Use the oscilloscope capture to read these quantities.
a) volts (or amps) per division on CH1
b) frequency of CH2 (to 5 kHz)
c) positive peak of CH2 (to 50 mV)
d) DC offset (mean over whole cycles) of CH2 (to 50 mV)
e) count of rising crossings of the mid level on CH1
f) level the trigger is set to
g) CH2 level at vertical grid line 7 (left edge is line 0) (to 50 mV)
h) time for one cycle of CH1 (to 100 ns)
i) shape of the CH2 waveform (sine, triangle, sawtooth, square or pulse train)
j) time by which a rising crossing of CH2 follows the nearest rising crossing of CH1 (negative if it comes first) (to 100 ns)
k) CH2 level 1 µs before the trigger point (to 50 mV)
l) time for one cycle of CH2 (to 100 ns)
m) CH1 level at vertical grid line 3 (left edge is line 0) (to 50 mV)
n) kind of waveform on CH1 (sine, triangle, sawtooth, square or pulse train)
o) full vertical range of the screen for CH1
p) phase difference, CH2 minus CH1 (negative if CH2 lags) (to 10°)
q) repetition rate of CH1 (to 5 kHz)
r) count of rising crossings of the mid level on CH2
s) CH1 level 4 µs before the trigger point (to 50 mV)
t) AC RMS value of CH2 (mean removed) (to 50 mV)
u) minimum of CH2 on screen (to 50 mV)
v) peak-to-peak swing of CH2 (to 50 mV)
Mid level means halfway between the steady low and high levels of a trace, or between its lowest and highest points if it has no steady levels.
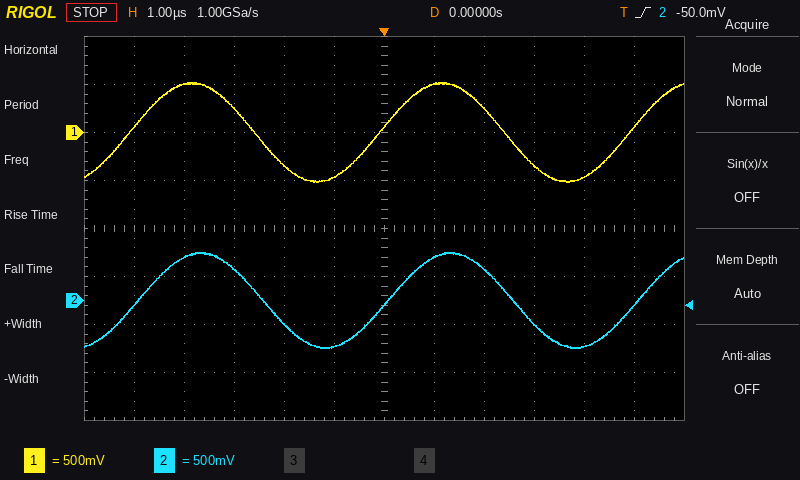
500 mV
200 kHz
500 mV
0 mV
3
-50.0 mV
450 mV
5.0 µs
sine
+200 ns
-500 mV
5.0 µs
250 mV
sine
4 V
-10°
200 kHz
3
500 mV
350 mV
-500 mV
1.00 V
